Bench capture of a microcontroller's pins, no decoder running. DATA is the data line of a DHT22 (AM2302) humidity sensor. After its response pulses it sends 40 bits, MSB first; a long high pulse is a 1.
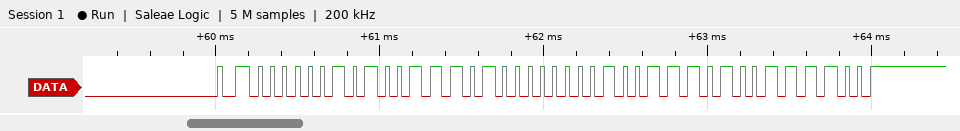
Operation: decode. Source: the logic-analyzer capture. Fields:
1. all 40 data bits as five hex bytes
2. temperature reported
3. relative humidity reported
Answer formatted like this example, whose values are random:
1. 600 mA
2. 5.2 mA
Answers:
1. 02 9D 00 9D 3C
2. 15.7 °C
3. 66.9 %
